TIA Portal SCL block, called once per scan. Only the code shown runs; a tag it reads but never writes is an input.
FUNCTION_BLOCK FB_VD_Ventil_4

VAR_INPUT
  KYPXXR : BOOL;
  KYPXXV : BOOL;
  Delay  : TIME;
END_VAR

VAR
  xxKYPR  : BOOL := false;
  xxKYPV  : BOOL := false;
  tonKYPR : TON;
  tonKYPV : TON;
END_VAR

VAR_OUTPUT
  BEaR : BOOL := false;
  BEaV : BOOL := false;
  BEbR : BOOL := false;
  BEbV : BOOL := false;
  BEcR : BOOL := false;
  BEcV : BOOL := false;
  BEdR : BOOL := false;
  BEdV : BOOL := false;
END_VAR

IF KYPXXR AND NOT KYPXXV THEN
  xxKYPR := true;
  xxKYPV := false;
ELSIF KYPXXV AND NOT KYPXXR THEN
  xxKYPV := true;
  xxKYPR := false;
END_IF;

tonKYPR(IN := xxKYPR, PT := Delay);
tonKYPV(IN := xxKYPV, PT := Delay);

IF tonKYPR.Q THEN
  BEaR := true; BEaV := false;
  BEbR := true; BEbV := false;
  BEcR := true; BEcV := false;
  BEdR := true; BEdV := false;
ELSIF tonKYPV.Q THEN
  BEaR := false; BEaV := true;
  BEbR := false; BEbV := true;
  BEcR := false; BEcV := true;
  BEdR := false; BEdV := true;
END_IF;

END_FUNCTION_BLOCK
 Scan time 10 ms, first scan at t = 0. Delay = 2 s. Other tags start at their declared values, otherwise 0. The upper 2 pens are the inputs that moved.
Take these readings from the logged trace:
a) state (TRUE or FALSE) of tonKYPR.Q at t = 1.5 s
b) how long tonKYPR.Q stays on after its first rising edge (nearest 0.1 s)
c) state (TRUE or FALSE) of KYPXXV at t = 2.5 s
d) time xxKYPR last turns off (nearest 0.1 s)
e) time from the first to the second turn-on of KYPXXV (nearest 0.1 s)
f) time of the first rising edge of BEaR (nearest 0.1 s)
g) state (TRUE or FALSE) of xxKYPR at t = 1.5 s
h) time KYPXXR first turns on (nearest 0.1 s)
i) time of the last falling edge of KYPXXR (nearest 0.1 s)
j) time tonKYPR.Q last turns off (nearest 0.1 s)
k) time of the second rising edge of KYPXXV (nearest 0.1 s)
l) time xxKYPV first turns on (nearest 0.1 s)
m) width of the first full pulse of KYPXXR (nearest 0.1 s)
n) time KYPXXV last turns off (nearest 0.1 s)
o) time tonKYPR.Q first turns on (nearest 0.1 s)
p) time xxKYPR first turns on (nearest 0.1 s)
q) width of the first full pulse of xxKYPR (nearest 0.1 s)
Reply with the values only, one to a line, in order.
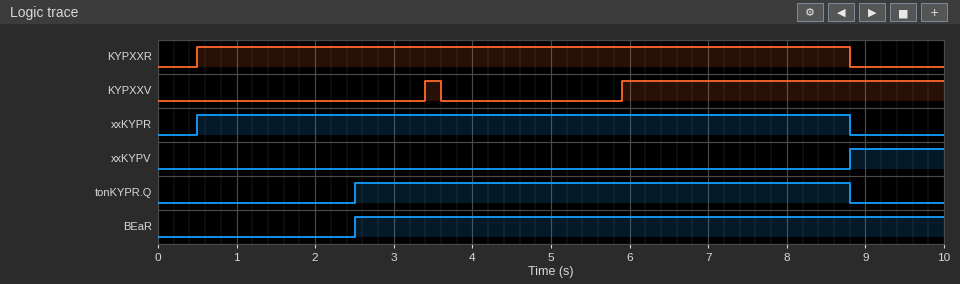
FALSE
6.3 s
FALSE
8.8 s
2.5 s
2.5 s
TRUE
0.5 s
8.8 s
8.8 s
5.9 s
8.8 s
8.3 s
3.6 s
2.5 s
0.5 s
8.3 s
